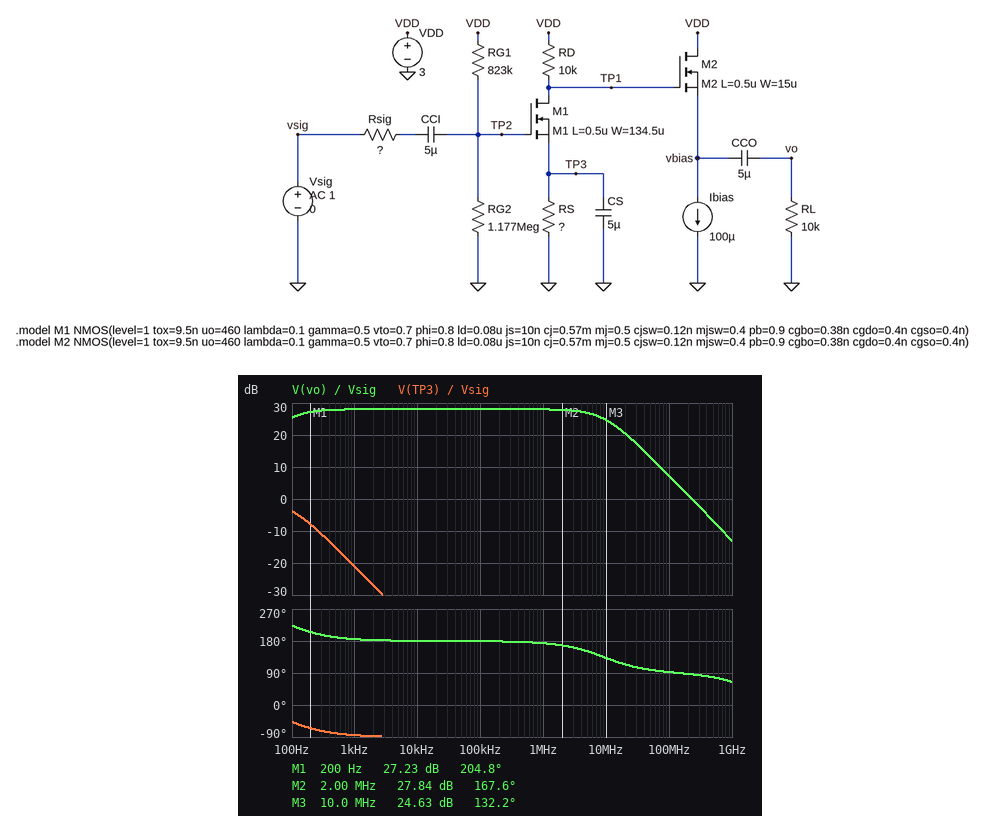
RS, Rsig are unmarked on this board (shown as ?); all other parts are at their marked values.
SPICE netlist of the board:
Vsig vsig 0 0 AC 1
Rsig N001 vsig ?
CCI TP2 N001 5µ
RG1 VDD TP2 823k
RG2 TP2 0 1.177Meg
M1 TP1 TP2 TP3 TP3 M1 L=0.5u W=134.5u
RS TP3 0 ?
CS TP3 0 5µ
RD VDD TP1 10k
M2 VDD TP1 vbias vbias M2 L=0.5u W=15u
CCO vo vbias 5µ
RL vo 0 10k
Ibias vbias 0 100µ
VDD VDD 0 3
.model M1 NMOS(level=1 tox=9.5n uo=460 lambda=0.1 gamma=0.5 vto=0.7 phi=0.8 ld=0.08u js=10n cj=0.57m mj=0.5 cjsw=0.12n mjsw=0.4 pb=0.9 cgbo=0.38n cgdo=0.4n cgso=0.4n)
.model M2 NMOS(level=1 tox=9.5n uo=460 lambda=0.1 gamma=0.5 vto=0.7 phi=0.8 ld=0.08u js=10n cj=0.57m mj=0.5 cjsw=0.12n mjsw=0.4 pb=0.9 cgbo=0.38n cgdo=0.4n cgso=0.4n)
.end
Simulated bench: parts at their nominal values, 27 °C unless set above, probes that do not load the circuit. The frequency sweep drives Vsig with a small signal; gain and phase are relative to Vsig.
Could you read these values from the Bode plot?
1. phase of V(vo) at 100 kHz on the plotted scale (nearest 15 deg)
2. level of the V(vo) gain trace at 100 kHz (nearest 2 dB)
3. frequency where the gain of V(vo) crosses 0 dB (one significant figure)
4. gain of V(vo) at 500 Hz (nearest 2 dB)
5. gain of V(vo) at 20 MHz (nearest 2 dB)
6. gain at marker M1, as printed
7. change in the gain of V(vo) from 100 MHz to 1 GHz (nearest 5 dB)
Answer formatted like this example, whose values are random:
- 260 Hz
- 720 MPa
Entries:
- 180 deg
- 28 dB
- 200 MHz
- 28 dB
- 20 dB
- 27.23 dB
- -20 dB
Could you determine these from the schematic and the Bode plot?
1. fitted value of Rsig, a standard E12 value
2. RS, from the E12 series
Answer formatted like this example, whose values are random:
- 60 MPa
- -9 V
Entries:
- 10 kΩ
- 18 kΩ
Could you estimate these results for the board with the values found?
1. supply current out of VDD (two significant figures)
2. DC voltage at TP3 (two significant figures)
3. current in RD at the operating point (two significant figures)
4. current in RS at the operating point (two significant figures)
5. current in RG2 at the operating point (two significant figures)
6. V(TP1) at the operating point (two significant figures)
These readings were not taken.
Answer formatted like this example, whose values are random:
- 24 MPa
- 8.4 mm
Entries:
- 160 µA
- 1.0 V
- 57 µA
- 57 µA
- 1.5 µA
- 2.4 V
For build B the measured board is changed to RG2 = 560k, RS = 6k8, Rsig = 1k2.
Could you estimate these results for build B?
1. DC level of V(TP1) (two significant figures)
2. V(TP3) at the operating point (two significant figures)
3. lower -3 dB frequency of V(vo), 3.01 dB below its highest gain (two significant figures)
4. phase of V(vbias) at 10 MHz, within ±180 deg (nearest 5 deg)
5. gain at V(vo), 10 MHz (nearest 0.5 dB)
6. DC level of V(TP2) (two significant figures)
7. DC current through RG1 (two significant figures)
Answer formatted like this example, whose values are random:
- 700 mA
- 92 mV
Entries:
- 2.3 V
- 470 mV
- 100 Hz
- 170 deg
- 29.0 dB
- 1.2 V
- 2.2 µA
